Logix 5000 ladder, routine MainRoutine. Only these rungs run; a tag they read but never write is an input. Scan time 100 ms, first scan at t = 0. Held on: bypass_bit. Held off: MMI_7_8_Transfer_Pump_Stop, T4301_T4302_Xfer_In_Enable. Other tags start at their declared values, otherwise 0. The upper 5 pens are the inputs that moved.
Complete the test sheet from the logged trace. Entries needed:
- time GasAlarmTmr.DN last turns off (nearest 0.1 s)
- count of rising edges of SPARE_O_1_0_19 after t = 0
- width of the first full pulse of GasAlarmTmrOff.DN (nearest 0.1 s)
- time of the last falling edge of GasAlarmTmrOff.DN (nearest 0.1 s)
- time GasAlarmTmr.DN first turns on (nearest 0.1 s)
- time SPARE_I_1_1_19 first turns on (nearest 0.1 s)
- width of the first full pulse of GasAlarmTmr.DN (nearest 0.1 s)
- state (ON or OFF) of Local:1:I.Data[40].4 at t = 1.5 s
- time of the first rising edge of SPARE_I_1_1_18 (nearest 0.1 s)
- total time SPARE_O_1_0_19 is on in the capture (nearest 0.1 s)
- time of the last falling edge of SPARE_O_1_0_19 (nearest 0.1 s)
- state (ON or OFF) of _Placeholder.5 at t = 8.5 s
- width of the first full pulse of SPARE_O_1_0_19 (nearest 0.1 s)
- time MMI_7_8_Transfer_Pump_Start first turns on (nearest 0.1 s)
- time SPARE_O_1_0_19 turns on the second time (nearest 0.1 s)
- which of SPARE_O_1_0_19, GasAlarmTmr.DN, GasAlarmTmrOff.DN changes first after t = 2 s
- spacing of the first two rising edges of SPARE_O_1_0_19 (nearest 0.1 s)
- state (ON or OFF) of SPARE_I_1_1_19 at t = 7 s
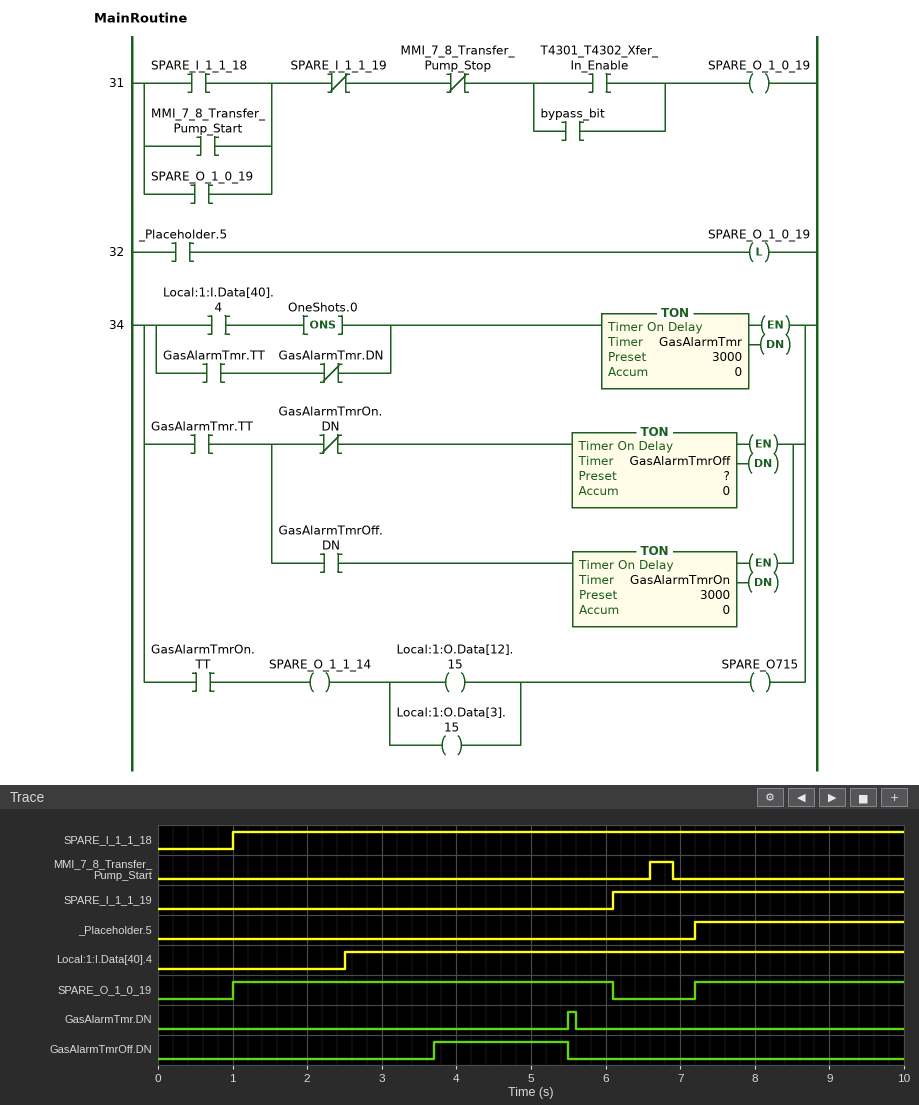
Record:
5.6 s
2
1.8 s
5.5 s
5.5 s
6.1 s
0.1 s
OFF
1.0 s
7.9 s
6.1 s
ON
5.1 s
6.6 s
7.2 s
GasAlarmTmrOff.DN
6.2 s
ON
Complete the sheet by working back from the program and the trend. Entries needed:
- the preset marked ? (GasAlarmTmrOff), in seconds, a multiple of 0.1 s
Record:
1.2 s
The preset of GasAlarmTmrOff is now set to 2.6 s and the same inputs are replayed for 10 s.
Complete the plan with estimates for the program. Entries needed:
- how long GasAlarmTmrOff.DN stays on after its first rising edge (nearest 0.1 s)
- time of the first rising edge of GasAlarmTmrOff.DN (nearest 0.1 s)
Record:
0.4 s
5.1 s
